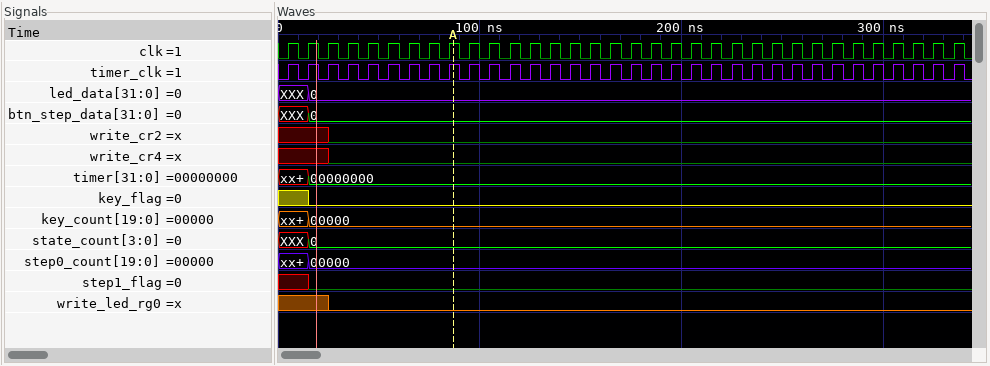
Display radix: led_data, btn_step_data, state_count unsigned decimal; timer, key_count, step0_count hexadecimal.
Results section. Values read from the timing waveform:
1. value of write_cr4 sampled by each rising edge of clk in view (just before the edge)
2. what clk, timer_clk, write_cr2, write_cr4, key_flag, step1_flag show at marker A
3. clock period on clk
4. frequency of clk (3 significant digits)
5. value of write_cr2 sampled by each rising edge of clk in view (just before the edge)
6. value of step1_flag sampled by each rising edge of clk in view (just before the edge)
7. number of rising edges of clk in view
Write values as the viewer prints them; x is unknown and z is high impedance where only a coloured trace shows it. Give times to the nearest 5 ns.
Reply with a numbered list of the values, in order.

1. x x x 0 0 0 0 0 0 0 0 0 0 0 0 0 0 0 0 0 0 0 0 0 0 0 0 0 0 0 0 0 0 0
2. clk=1, timer_clk=1, write_cr2=0, write_cr4=0, key_flag=0, step1_flag=0
3. 10 ns
4. 100 MHz
5. x x x 0 0 0 0 0 0 0 0 0 0 0 0 0 0 0 0 0 0 0 0 0 0 0 0 0 0 0 0 0 0 0
6. x x 0 0 0 0 0 0 0 0 0 0 0 0 0 0 0 0 0 0 0 0 0 0 0 0 0 0 0 0 0 0 0 0
7. 34
